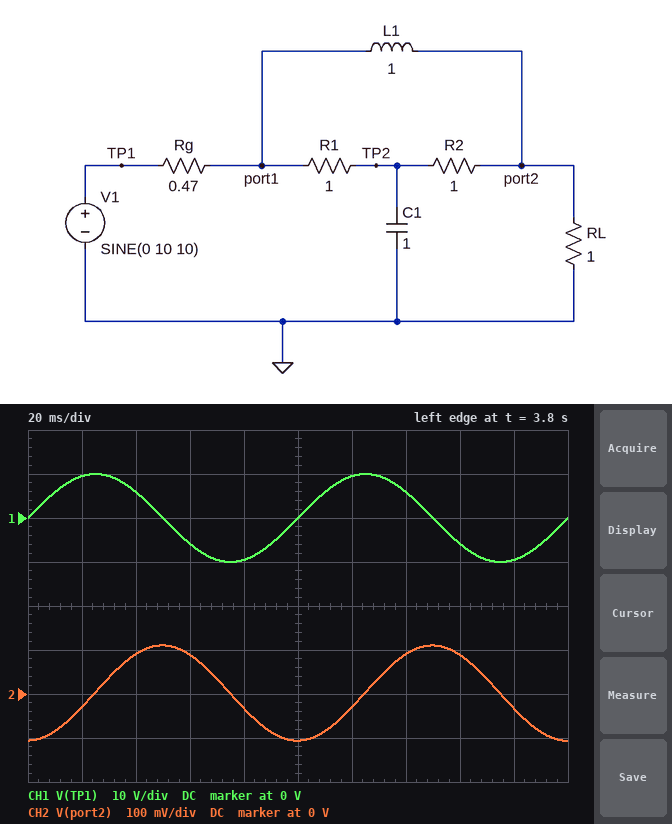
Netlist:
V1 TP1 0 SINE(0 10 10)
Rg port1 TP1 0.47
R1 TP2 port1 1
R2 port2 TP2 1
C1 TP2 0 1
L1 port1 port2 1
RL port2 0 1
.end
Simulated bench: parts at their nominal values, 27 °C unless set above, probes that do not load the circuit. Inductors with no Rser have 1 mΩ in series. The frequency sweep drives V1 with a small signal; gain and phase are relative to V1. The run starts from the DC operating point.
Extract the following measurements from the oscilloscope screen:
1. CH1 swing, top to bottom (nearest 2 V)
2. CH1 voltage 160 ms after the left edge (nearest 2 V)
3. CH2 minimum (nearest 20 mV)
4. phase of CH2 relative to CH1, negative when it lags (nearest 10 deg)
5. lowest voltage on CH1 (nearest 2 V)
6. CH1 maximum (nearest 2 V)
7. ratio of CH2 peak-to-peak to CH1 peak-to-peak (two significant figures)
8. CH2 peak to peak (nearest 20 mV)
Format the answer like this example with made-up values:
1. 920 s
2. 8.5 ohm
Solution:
1. 20 V
2. -6 V
3. -100 mV
4. -90 deg
5. -10 V
6. 10 V
7. 0.011
8. 220 mV
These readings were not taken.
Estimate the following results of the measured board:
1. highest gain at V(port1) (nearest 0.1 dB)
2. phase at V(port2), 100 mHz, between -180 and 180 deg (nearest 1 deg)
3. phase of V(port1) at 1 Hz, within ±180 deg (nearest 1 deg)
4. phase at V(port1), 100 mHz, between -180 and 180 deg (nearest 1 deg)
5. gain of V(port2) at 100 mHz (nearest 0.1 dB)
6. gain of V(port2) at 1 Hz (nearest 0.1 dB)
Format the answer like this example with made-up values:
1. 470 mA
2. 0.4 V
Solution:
1. -3.3 dB
2. -32 deg
3. 0 deg
4. 0 deg
5. -4.8 dB
6. -19.4 dB
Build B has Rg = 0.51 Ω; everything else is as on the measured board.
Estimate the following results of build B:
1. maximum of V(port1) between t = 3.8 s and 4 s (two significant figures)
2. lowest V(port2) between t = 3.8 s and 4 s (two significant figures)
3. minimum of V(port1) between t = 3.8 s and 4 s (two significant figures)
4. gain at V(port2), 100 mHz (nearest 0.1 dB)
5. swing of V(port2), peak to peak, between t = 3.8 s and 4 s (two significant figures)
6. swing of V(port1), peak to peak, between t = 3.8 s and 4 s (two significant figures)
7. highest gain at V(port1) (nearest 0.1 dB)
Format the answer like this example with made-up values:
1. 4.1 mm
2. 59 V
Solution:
1. 6.6 V
2. -100 mV
3. -6.6 V
4. -5.0 dB
5. 210 mV
6. 13 V
7. -3.6 dB
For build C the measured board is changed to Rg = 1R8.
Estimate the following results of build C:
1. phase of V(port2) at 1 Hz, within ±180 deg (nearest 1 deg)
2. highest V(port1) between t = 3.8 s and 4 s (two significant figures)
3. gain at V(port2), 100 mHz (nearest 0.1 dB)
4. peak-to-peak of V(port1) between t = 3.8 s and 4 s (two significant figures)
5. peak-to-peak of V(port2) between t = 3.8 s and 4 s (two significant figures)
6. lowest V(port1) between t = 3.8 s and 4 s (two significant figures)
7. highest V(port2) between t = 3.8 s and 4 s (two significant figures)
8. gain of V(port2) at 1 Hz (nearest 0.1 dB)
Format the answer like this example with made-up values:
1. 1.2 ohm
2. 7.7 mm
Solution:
1. -81 deg
2. 3.6 V
3. -10.4 dB
4. 7.1 V
5. 110 mV
6. -3.6 V
7. 58 mV
8. -25.0 dB
